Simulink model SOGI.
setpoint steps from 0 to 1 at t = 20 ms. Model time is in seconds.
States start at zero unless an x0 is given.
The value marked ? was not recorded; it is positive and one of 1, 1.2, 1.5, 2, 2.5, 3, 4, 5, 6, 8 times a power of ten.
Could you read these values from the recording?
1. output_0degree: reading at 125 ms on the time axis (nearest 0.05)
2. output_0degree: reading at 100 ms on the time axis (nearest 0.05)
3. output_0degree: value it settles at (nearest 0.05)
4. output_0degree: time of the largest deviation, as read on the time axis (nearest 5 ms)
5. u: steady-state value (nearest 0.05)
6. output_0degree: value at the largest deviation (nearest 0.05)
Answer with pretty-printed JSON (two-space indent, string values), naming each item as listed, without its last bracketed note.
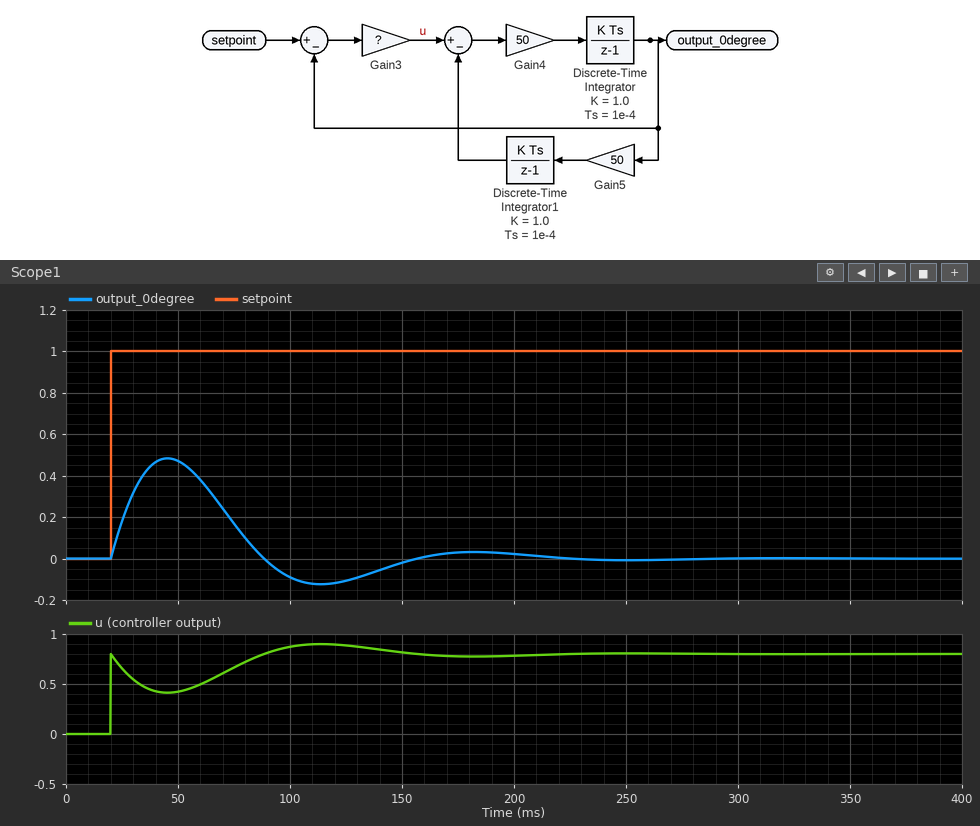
{
  "output_0degree: reading at 125 ms on the time axis": "-0.10",
  "output_0degree: reading at 100 ms on the time axis": "-0.10",
  "output_0degree: value it settles at": "0.00",
  "output_0degree: time of the largest deviation, as read on the time axis": "45 ms",
  "u: steady-state value": "0.80",
  "output_0degree: value at the largest deviation": "0.50"
}
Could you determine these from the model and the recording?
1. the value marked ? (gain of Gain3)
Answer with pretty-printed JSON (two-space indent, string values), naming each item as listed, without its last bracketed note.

{
  "the value marked ?": "0.8"
}
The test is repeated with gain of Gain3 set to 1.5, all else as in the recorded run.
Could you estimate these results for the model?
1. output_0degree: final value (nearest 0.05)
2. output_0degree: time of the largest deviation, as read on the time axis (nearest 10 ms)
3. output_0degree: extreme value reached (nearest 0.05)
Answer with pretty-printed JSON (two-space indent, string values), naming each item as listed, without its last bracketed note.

{
  "output_0degree: final value": "0.00",
  "output_0degree: time of the largest deviation, as read on the time axis": "40 ms",
  "output_0degree: extreme value reached": "0.65"
}
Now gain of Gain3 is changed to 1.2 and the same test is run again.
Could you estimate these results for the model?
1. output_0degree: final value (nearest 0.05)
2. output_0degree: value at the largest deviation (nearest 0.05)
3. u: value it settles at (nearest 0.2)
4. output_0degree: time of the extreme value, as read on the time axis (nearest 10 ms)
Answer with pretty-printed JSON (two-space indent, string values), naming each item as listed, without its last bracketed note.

{
  "output_0degree: final value": "0.00",
  "output_0degree: value at the largest deviation": "0.60",
  "u: value it settles at": "1.2",
  "output_0degree: time of the extreme value, as read on the time axis": "40 ms"
}
